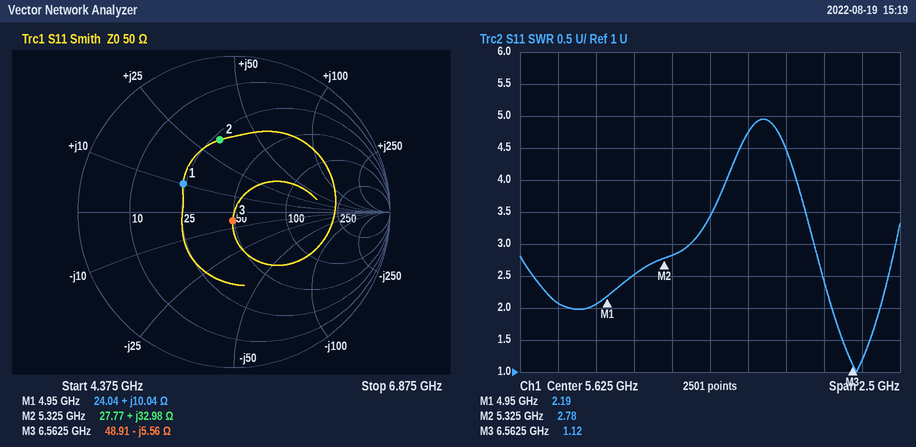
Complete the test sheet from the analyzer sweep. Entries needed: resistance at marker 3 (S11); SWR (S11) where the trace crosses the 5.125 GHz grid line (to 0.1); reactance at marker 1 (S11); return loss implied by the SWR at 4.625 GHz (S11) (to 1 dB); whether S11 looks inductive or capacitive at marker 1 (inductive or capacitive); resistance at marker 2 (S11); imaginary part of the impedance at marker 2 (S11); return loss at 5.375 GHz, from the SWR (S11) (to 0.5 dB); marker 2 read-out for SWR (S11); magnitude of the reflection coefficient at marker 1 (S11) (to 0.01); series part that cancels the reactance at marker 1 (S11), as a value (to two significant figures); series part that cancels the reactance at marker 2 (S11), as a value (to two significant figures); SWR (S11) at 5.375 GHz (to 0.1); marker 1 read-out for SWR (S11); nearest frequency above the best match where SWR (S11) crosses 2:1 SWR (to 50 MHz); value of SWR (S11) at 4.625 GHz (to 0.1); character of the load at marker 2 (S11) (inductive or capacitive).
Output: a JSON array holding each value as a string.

["48.91 Ω", "2.5", "+10.04 Ω", "9 dB", "inductive", "27.77 Ω", "+32.98 Ω", "6.5 dB", "2.78", "0.37", "3.2 pF", "910 fF", "2.8", "2.19", "6.75 GHz", "2.1", "inductive"]
